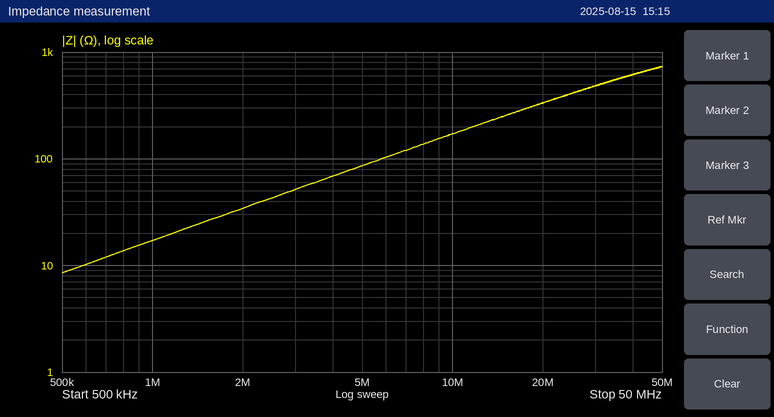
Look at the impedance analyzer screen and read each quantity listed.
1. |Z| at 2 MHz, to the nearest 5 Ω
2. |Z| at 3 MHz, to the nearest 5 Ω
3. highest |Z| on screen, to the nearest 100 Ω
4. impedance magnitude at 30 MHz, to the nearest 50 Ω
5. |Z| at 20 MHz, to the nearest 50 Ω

35 Ω
50 Ω
700 Ω
500 Ω
350 Ω
